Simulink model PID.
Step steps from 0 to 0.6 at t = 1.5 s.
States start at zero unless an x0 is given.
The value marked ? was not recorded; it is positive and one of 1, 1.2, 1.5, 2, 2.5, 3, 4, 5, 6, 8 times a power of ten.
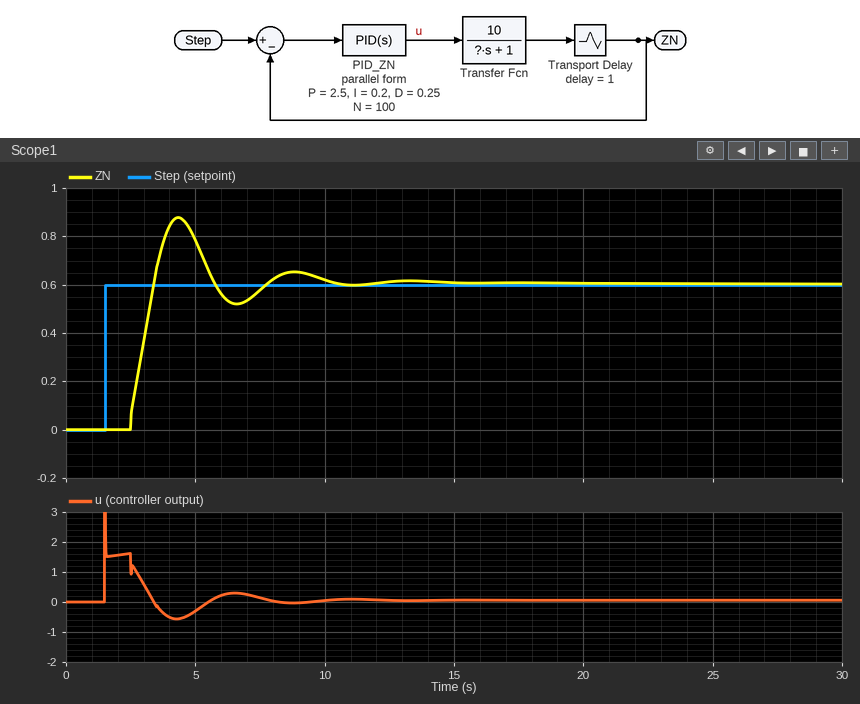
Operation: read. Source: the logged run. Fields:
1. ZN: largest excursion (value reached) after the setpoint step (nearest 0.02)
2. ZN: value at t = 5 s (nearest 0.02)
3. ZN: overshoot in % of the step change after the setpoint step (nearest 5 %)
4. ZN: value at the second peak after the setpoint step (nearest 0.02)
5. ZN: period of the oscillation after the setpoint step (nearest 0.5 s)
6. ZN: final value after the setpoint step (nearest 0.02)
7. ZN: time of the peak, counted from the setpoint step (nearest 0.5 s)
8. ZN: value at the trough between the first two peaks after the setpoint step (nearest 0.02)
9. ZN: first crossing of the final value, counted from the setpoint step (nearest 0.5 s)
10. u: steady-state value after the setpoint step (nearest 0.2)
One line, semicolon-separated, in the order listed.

0.88; 0.78; 45 %; 0.66; 4.5 s; 0.60; 3.0 s; 0.52; 2.0 s; 0.0
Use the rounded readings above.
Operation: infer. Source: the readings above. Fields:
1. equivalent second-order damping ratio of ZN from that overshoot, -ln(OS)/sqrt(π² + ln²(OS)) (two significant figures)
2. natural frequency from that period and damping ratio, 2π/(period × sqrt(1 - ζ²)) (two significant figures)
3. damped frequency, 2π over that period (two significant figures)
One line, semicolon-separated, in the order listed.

0.25; 1.4 rad/s; 1.4 rad/s
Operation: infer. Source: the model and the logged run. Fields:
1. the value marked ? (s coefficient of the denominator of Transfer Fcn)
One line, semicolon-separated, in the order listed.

25
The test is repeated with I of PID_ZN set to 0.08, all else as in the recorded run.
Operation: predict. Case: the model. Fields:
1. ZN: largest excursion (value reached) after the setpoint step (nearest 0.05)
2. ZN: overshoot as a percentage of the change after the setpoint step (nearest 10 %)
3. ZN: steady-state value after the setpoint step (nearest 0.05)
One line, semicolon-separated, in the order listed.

0.85; 40 %; 0.60
